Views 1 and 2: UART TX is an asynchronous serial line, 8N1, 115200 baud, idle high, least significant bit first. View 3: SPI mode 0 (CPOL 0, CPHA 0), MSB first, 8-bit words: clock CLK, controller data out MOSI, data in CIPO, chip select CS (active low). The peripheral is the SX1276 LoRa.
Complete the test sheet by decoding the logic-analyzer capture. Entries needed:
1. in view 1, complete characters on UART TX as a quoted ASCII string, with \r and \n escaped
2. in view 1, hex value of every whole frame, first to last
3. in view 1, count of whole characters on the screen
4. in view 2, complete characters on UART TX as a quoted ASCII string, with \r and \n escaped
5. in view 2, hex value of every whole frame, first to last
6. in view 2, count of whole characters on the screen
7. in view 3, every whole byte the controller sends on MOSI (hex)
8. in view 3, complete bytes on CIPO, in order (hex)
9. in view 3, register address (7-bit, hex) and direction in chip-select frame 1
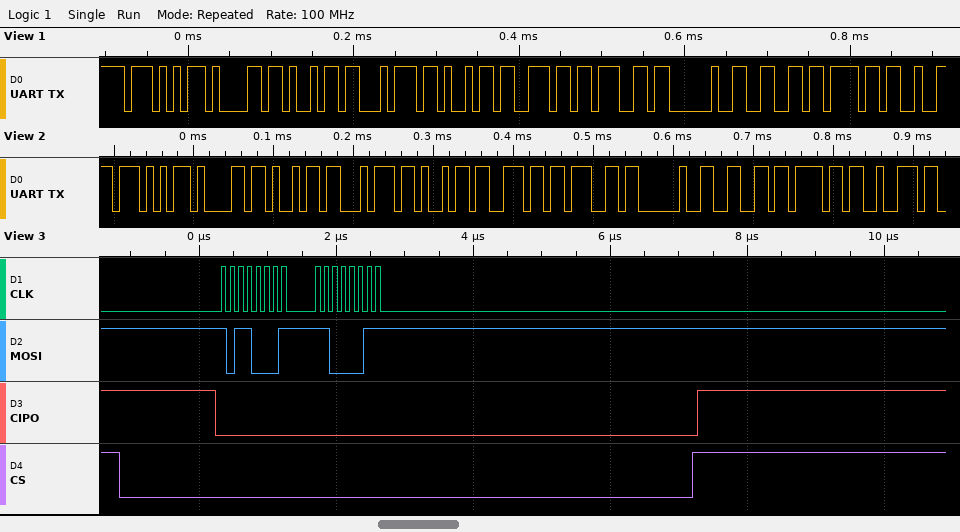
"Waiting fo"
57 61 69 74 69 6E 67 20 66 6F
10
"Waiting for"
57 61 69 74 69 6E 67 20 66 6F 72
11
B1 C3
00 00
0x31 write
